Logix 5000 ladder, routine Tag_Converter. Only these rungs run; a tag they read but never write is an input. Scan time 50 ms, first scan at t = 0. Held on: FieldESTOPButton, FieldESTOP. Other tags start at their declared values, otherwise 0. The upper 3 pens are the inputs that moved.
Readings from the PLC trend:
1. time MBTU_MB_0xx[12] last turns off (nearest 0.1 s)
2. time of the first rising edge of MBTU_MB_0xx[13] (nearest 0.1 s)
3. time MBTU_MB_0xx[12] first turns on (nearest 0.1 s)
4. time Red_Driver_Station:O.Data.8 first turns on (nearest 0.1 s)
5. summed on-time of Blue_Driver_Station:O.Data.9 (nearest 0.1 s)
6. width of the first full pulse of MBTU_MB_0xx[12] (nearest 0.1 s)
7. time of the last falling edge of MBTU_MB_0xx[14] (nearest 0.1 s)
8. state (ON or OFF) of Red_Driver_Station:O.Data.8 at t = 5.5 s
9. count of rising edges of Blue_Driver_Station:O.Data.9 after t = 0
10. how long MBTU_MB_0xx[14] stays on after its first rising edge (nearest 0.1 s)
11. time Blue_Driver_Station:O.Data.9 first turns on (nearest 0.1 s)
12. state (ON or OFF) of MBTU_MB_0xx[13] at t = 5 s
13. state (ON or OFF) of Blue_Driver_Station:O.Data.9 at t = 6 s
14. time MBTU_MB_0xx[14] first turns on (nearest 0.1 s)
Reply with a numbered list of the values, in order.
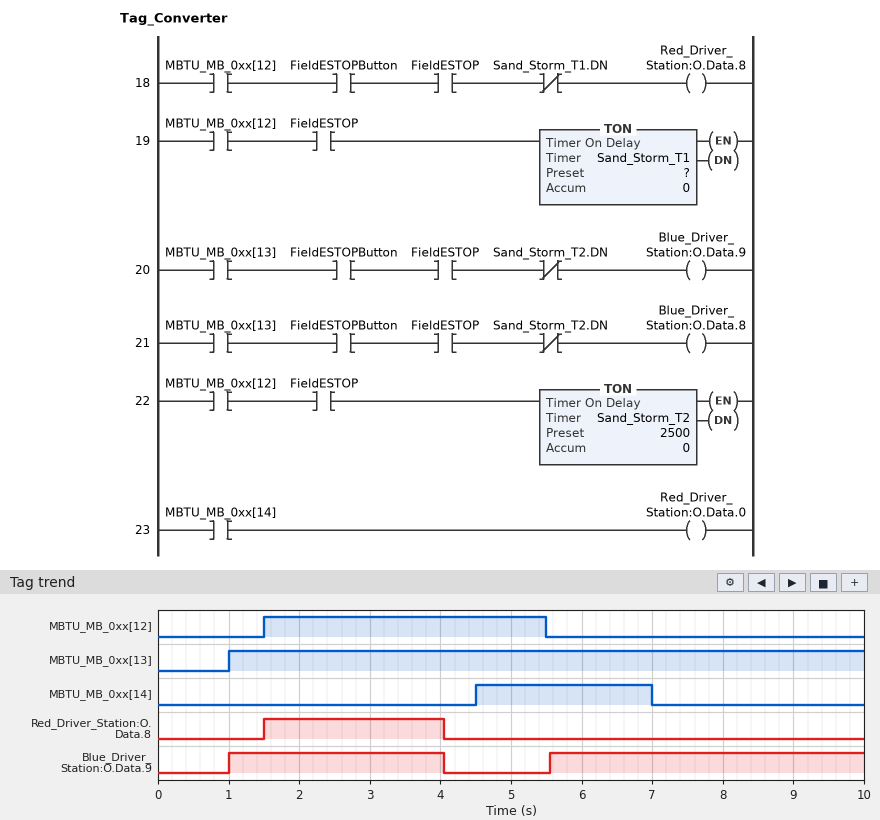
1. 5.5 s
2. 1.0 s
3. 1.5 s
4. 1.5 s
5. 7.5 s
6. 4.0 s
7. 7.0 s
8. OFF
9. 2
10. 2.5 s
11. 1.0 s
12. ON
13. ON
14. 4.5 s
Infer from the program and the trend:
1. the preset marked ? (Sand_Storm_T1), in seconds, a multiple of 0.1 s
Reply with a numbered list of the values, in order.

1. 2.5 s
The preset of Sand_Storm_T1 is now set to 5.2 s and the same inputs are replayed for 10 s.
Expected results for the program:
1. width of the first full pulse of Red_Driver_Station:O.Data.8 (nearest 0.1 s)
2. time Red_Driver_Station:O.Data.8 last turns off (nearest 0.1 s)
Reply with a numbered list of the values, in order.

1. 4.0 s
2. 5.5 s
